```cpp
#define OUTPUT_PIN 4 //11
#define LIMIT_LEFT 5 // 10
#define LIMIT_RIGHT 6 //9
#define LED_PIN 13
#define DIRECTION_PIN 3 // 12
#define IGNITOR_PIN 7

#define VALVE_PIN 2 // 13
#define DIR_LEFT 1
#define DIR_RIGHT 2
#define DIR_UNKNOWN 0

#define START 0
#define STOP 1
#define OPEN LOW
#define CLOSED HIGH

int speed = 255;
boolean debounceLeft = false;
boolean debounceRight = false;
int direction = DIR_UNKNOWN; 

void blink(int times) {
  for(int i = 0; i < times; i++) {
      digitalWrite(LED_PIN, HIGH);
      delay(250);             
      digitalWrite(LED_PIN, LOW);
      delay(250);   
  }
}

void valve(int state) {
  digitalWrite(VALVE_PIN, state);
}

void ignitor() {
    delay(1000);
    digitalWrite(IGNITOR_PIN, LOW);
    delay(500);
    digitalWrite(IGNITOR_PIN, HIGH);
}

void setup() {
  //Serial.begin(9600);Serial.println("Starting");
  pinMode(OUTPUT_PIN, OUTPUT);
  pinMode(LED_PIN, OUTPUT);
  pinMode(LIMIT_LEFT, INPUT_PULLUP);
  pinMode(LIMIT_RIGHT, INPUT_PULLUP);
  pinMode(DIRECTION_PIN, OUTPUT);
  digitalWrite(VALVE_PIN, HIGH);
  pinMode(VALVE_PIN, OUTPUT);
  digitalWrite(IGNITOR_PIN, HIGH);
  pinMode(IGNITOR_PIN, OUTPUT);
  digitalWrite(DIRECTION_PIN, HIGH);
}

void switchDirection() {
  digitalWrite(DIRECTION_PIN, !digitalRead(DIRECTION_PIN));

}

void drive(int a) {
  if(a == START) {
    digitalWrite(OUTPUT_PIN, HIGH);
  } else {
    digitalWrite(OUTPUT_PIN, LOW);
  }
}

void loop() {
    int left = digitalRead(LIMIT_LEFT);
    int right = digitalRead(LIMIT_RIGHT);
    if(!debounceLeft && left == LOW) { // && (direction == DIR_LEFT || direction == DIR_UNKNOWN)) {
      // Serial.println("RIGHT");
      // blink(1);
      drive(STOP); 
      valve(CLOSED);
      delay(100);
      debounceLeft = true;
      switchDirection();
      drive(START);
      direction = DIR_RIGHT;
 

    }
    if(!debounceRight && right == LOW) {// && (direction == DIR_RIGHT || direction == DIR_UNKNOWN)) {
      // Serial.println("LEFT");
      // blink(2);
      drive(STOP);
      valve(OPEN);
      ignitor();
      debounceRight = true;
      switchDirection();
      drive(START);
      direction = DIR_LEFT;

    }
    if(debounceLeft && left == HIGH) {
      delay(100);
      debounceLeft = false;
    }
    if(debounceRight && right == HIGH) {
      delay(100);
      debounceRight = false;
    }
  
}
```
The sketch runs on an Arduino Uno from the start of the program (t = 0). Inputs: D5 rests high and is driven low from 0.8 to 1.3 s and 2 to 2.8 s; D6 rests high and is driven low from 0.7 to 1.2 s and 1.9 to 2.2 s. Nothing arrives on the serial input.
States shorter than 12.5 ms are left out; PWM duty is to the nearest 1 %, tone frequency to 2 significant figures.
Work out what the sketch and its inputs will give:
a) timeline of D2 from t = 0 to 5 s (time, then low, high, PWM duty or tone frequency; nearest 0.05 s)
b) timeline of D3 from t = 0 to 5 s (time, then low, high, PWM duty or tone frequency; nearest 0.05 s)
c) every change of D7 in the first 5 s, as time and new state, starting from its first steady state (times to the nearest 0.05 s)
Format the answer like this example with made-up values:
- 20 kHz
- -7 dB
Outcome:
- 0 s high; 0.7 s low; 2.2 s high
- 0 s high; 2.2 s low; 2.3 s high
- 0 s high; 1.7 s low; 2.2 s high
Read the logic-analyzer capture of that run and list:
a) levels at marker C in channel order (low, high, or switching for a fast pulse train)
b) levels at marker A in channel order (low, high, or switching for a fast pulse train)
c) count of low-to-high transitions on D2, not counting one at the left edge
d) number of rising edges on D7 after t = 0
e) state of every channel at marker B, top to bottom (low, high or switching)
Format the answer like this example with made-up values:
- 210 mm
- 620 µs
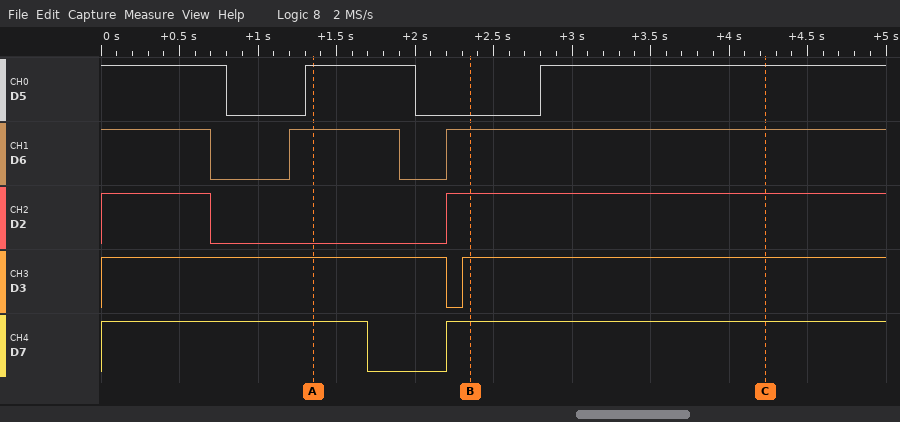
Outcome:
- D5 high, D6 high, D2 high, D3 high, D7 high
- D5 high, D6 high, D2 low, D3 high, D7 high
- 1
- 1
- D5 low, D6 high, D2 high, D3 high, D7 high
